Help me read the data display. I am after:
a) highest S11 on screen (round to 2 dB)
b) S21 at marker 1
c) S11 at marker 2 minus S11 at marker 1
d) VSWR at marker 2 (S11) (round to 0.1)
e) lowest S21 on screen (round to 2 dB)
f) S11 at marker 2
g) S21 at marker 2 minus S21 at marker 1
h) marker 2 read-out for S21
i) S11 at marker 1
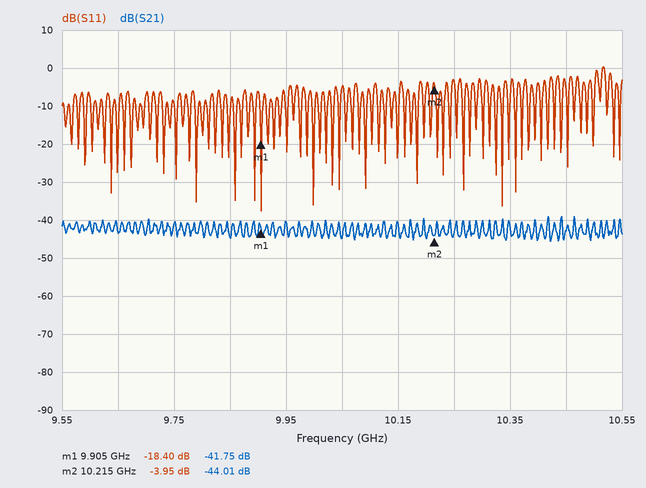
0 dB
-41.75 dB
14.45 dB
4.5
-46 dB
-3.95 dB
-2.26 dB
-44.01 dB
-18.40 dB
